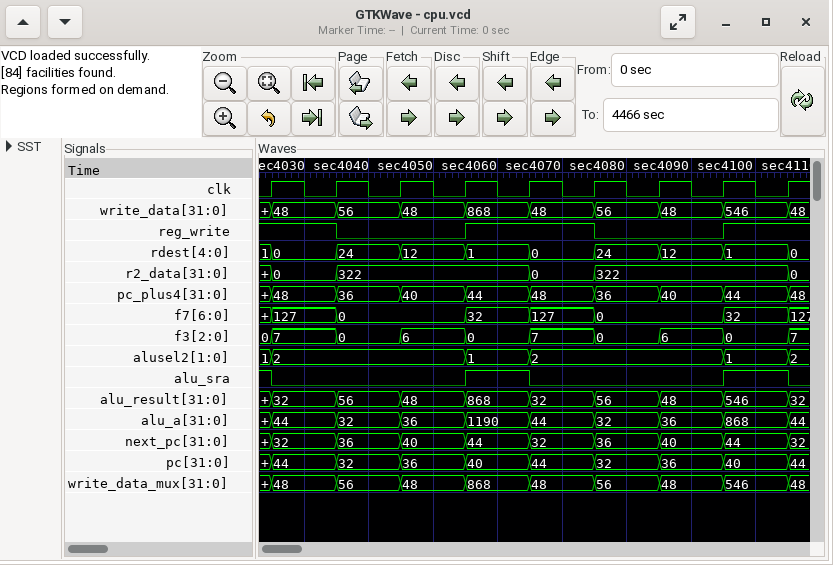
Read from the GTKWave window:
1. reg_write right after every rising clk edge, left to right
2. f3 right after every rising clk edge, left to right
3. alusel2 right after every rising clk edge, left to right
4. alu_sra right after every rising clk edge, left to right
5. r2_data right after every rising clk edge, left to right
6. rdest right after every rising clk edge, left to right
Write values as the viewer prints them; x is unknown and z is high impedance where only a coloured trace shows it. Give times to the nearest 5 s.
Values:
1 0 0 1 1 0 0 1 1
7, 0, 6, 0, 7, 0, 6, 0, 7
2, 2, 2, 1, 2, 2, 2, 1, 2
0 0 0 1 0 0 0 1 0
0, 322, 322, 322, 0, 322, 322, 322, 0
0, 24, 12, 1, 0, 24, 12, 1, 0
